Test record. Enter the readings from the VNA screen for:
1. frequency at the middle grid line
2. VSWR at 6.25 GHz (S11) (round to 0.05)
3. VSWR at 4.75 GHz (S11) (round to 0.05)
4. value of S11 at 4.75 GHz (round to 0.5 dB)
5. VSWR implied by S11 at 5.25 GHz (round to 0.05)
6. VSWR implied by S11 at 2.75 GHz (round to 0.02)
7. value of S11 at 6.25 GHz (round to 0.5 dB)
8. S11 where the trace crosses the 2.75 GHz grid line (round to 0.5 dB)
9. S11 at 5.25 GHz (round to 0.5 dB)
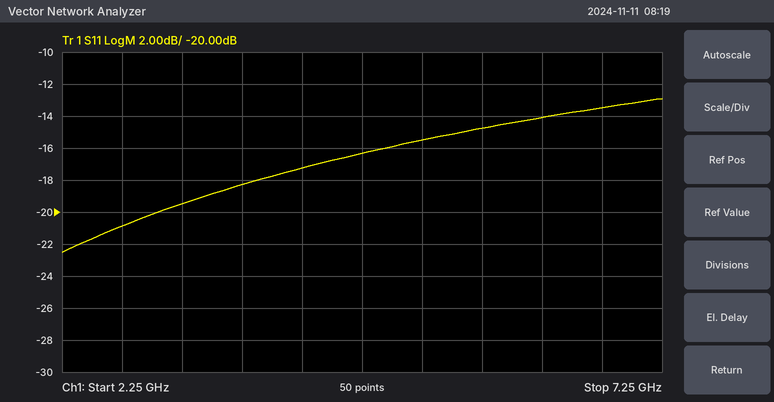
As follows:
4.75 GHz
1.50
1.35
-16.5 dB
1.40
1.20
-14.0 dB
-21.0 dB
-15.5 dB
